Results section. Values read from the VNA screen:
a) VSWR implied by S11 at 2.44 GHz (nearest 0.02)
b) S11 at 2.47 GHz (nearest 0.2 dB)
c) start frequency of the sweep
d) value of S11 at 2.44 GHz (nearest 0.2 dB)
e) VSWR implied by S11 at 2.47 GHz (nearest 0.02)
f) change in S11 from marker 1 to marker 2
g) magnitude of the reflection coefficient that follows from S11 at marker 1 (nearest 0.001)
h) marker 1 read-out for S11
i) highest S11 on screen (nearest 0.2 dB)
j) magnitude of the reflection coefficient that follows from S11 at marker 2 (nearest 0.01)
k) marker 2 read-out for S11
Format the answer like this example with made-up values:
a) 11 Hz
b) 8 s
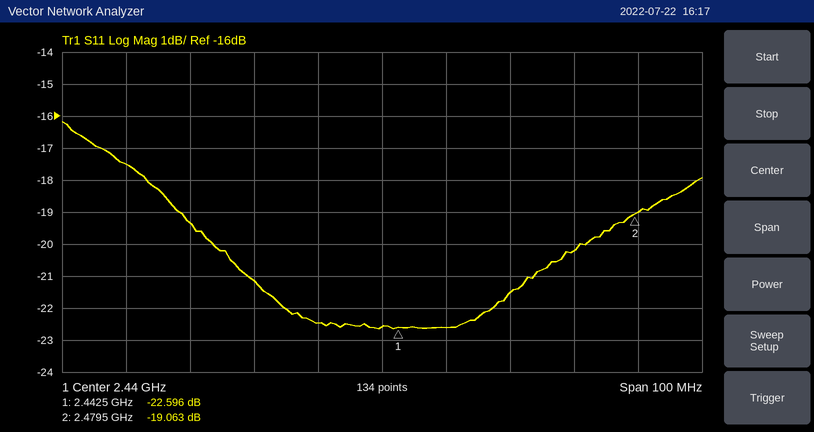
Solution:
a) 1.16
b) -20.2 dB
c) 2.39 GHz
d) -22.6 dB
e) 1.22
f) 3.533 dB
g) 0.074
h) -22.596 dB
i) -16.2 dB
j) 0.11
k) -19.063 dB
